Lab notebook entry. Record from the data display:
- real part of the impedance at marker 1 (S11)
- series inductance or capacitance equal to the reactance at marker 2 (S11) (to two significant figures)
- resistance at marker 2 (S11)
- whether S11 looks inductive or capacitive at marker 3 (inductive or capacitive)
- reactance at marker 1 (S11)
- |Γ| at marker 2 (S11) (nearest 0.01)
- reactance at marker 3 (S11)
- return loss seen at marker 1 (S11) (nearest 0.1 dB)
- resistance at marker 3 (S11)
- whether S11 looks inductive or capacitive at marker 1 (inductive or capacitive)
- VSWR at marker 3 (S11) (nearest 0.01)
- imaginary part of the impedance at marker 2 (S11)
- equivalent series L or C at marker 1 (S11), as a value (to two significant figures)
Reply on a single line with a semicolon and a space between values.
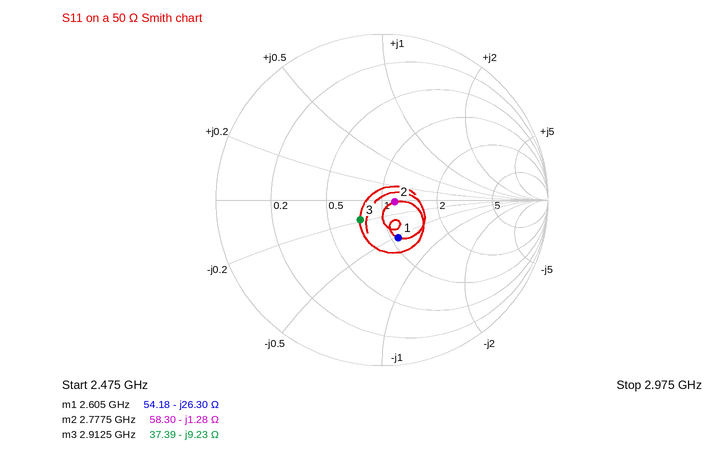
54.18 Ω; 45 pF; 58.30 Ω; capacitive; -26.30 Ω; 0.08; -9.23 Ω; 12.1 dB; 37.39 Ω; capacitive; 1.43; -1.28 Ω; 2.3 pF
